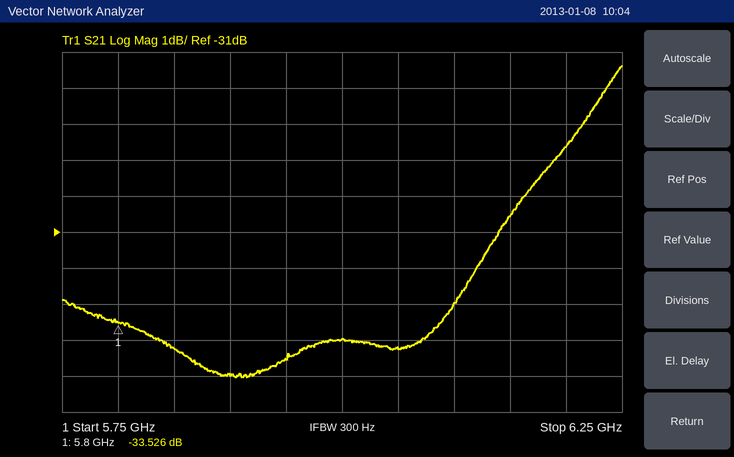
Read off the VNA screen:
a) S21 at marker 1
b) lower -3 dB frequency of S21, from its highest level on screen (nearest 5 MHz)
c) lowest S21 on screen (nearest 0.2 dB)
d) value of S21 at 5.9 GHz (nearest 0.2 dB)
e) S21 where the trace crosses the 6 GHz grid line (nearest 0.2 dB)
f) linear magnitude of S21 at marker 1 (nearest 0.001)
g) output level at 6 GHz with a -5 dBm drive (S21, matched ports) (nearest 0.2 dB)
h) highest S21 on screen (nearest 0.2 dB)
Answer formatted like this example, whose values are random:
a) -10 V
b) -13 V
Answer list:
a) -33.526 dB
b) 6.180 GHz
c) -35.0 dB
d) -35.0 dB
e) -34.0 dB
f) 0.021
g) -39.0 dBm
h) -26.4 dB
